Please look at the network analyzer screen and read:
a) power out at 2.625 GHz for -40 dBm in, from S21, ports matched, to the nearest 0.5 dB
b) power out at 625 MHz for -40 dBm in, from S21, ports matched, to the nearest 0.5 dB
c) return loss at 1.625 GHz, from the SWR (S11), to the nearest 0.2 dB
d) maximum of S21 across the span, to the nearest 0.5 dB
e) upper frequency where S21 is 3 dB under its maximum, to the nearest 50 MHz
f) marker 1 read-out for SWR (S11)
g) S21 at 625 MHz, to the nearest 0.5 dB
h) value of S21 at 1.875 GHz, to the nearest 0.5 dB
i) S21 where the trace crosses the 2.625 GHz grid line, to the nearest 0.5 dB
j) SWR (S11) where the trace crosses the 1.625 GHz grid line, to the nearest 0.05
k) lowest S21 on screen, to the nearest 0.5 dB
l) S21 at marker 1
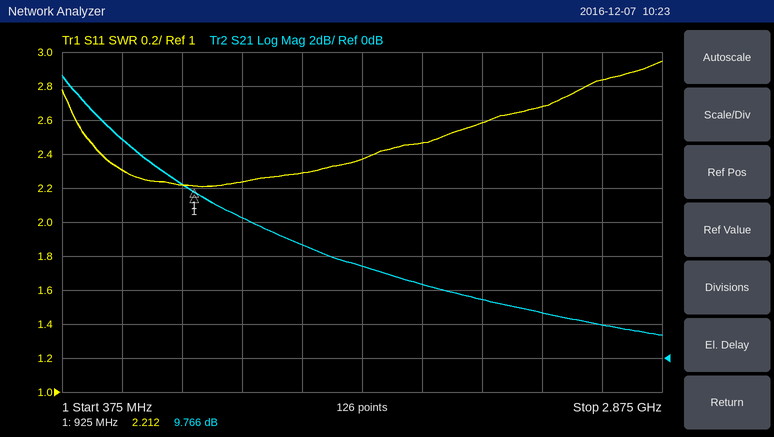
-38.0 dBm
-27.0 dBm
7.8 dB
16.5 dB
550 MHz
2.212
13.0 dB
4.5 dB
2.0 dB
2.35
1.5 dB
9.766 dB
